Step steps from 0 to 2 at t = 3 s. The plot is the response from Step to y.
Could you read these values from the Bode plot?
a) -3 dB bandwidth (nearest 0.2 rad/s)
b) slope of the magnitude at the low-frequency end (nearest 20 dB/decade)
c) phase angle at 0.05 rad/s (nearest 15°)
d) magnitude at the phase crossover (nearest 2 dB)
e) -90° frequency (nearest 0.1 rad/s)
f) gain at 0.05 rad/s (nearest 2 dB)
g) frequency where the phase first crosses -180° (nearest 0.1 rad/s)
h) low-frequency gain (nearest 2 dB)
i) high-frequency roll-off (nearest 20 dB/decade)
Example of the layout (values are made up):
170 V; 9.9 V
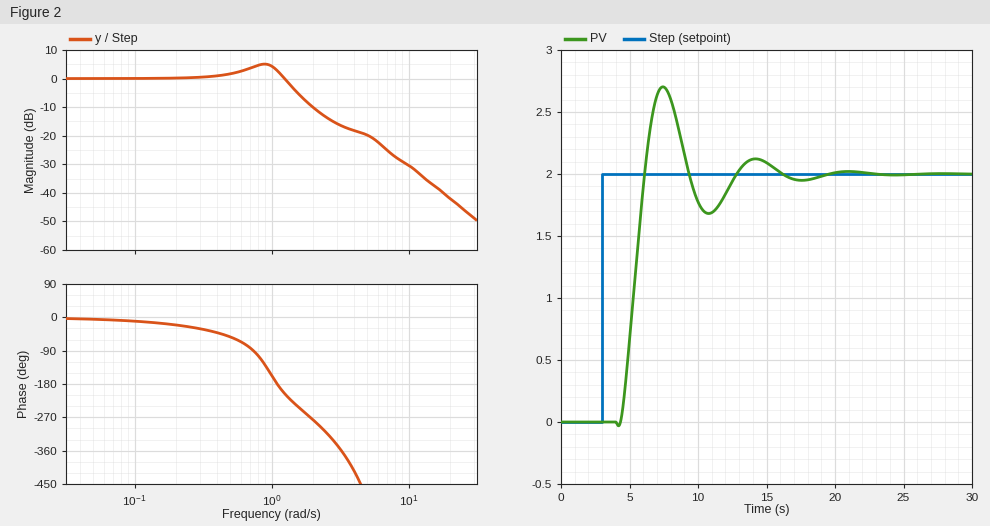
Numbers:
1.4 rad/s; 0 dB/decade; 0°; 2 dB; 0.7 rad/s; 0 dB; 1.1 rad/s; 0 dB; -40 dB/decade
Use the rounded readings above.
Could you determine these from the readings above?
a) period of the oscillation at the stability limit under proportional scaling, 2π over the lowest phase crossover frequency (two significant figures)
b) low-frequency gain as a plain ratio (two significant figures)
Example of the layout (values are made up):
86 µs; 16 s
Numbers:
5.7 s; 1.0
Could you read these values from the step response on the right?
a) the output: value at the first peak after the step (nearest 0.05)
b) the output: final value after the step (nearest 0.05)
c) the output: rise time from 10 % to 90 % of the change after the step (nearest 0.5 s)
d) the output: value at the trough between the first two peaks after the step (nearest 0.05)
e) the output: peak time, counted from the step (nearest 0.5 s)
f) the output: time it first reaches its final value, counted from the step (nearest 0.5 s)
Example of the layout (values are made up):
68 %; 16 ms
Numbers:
2.70; 2.00; 1.5 s; 1.70; 4.5 s; 3.0 s
